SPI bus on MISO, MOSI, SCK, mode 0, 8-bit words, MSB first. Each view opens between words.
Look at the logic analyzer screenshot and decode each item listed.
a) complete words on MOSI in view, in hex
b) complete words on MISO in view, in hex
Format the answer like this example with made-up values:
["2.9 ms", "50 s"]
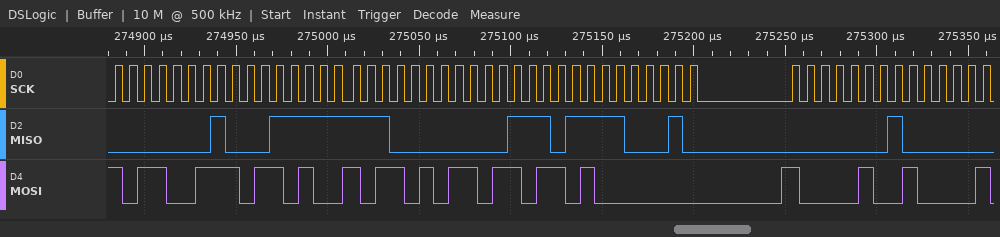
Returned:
["B3, B4, B5, B6, 80, 84", "01, 1F, E0, 1D, E2, 01"]
